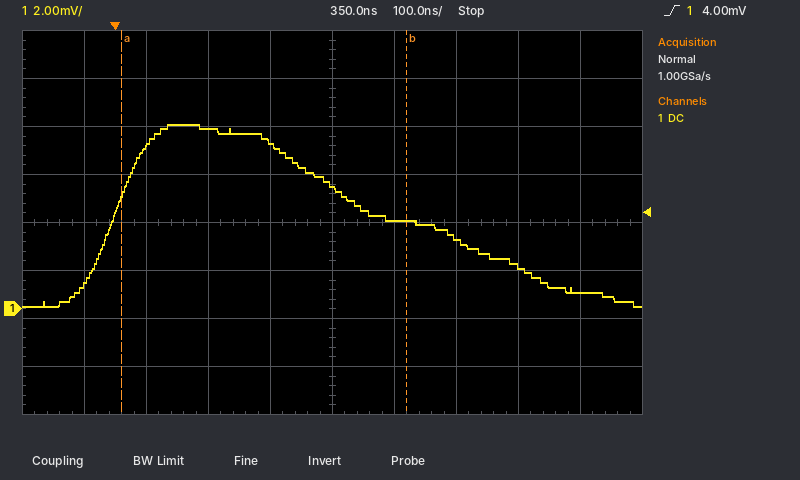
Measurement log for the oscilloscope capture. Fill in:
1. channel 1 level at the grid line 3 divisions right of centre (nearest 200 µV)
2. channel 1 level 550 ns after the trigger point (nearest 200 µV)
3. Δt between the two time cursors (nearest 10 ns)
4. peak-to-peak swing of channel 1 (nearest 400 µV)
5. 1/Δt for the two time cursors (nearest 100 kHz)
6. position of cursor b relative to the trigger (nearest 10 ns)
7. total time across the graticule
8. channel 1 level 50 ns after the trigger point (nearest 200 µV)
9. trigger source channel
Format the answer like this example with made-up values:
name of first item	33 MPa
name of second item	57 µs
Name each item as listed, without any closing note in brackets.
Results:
channel 1 level at the grid line 3 divisions right of centre	1.8 mV
channel 1 level 550 ns after the trigger point	3.0 mV
Δt between the two time cursors	460 ns
peak-to-peak swing of channel 1	7.6 mV
1/Δt for the two time cursors	2.2 MHz
position of cursor b relative to the trigger	+470 ns
total time across the graticule	1 µs
channel 1 level 50 ns after the trigger point	6.8 mV
trigger source channel	channel 1
